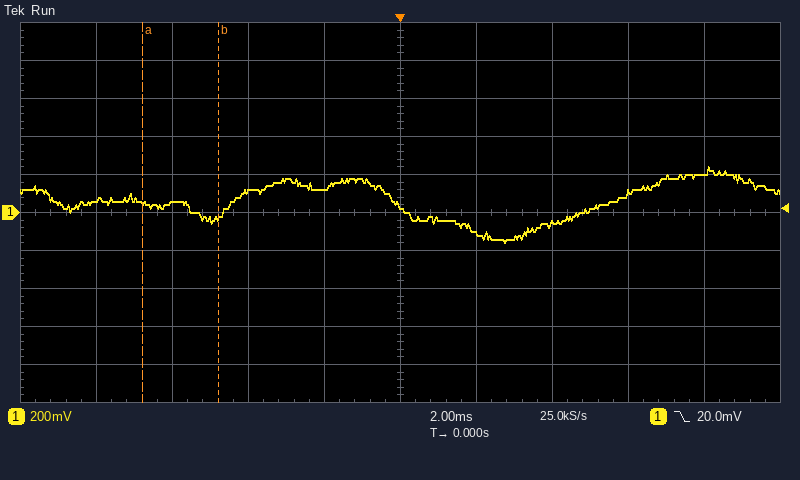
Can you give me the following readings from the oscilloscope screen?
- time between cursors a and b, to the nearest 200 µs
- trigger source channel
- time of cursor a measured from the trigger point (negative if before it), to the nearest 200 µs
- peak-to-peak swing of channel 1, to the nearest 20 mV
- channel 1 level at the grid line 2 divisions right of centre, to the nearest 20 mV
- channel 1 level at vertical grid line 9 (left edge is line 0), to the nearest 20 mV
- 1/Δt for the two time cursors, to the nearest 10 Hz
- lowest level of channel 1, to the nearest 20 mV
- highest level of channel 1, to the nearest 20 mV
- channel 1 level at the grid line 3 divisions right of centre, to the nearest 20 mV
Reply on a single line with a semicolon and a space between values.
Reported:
2.0 ms; channel 1; -6.8 ms; 400 mV; -60 mV; 220 mV; 500 Hz; -160 mV; 240 mV; 100 mV
